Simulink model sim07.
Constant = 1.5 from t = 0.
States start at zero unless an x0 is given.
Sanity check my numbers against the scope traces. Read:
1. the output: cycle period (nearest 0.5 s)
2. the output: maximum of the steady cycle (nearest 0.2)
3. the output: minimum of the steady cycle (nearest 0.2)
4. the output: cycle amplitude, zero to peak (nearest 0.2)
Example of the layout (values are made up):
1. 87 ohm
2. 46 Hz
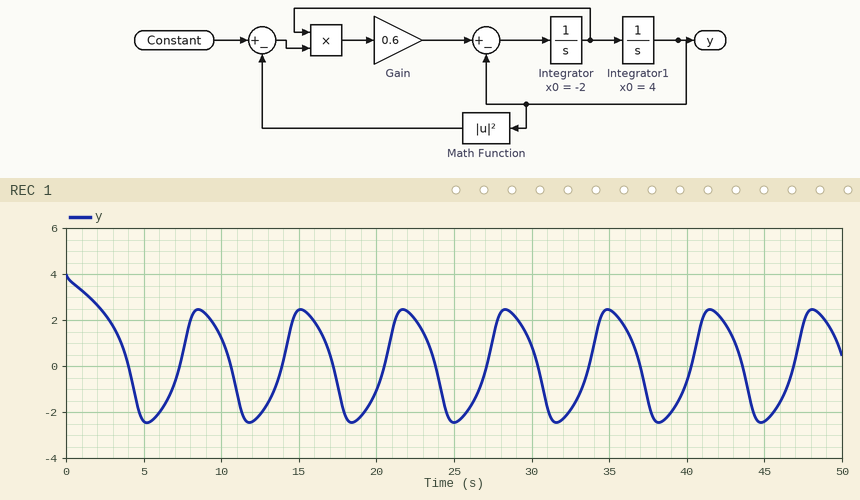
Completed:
1. 6.5 s
2. 2.4
3. -2.4
4. 2.4
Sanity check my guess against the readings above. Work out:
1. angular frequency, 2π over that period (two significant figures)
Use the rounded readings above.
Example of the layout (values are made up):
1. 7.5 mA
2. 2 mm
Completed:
1. 0.97 rad/s
